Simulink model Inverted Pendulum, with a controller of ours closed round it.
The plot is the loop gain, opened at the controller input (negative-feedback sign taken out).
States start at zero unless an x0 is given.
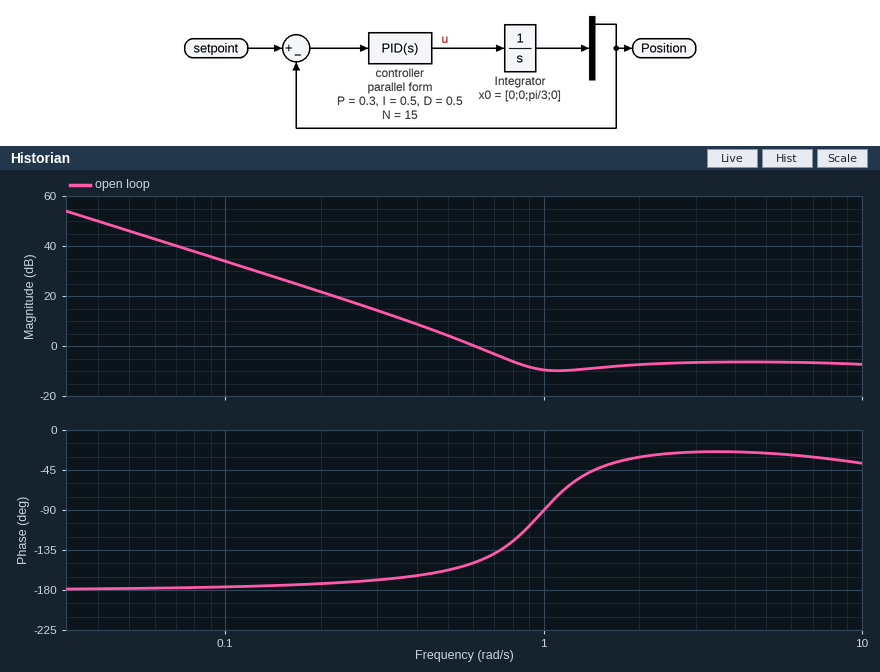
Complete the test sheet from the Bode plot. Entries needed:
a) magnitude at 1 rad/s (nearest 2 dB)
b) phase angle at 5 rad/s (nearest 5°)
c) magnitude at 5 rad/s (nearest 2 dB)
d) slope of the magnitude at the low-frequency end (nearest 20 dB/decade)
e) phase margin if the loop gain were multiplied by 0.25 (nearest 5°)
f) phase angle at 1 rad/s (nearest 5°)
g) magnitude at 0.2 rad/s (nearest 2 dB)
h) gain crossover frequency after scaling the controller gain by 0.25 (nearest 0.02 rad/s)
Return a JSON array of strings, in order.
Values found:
["-10 dB", "-25°", "-6 dB", "-40 dB/decade", "15°", "-90°", "22 dB", "0.34 rad/s"]
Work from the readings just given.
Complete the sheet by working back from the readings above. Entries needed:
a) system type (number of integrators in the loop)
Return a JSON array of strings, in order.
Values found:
["2"]
